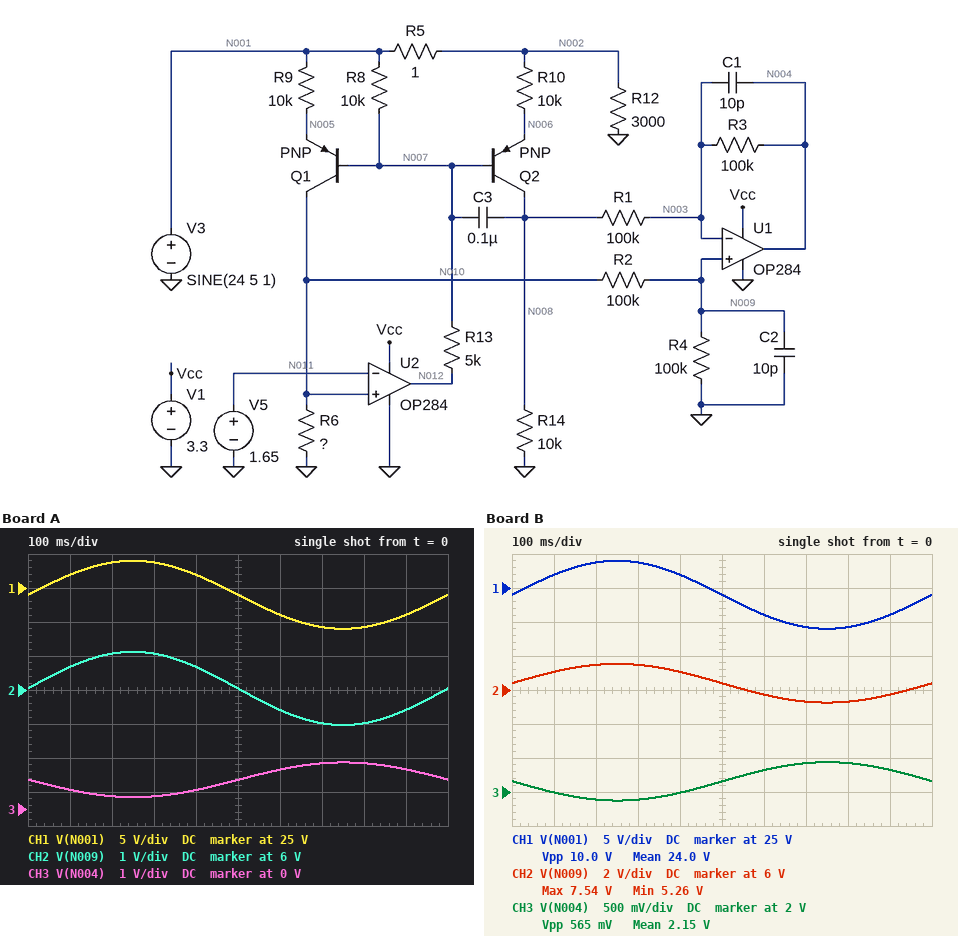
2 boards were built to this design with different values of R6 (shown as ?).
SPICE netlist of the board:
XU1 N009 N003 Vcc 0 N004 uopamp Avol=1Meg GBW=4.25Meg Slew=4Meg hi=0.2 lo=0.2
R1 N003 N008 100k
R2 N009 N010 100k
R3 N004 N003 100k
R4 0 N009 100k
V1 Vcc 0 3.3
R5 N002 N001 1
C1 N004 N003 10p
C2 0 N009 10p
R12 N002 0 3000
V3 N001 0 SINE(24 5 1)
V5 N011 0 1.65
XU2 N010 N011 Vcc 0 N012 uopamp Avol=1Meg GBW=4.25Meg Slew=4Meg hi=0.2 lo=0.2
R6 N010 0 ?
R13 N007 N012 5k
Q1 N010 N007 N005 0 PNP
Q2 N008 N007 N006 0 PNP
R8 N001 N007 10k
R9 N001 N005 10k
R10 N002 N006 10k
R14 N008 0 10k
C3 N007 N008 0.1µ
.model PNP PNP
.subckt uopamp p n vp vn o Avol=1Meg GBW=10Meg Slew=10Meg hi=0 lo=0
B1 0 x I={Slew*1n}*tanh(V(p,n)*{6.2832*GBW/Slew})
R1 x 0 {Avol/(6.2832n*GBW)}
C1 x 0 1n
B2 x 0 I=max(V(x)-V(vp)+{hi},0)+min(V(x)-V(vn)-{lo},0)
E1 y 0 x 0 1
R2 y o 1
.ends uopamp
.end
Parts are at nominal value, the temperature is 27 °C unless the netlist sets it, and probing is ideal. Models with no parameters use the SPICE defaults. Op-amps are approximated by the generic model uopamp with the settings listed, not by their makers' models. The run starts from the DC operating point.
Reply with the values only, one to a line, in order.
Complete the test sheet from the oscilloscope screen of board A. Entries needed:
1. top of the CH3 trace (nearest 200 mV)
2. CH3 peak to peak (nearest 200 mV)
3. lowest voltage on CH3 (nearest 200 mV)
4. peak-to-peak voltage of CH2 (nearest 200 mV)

1.4 V
1.0 V
400 mV
2.2 V
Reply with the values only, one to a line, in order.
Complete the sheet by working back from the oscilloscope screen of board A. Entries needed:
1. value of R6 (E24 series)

16 kΩ
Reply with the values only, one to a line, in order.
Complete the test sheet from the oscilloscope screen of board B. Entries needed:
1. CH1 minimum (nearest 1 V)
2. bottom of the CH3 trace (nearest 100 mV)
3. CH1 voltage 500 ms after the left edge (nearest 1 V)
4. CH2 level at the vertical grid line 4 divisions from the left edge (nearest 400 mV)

19 V
1.9 V
24 V
7.2 V
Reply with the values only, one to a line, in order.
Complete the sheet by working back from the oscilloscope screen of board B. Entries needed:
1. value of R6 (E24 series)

27 kΩ
